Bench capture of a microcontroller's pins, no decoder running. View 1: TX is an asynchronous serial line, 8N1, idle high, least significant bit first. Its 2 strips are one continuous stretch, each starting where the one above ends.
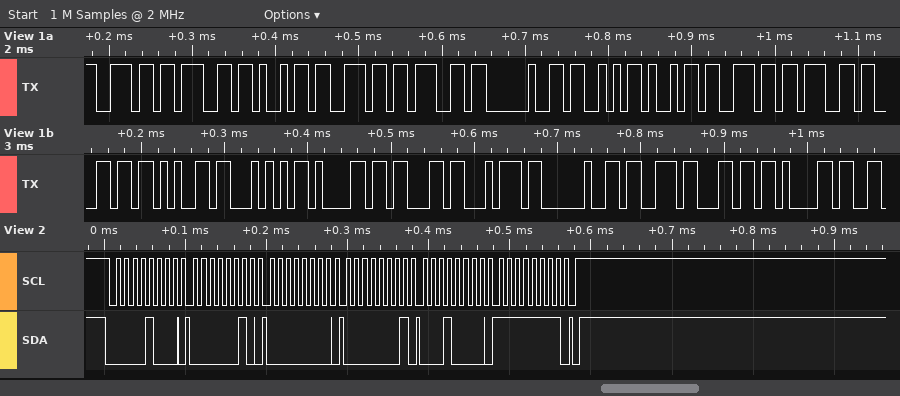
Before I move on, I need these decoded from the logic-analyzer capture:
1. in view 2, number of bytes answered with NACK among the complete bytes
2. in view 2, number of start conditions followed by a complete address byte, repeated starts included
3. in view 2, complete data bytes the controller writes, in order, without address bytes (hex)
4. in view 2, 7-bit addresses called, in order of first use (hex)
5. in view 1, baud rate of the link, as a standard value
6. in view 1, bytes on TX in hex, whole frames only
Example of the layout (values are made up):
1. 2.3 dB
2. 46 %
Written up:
1. 0
2. 1
3. 02 00 01 10 FF
4. 0x04
5. 115200 baud
6. 6E 67 69 6E 67 20 53 69 6E 67 6C 65 54 61 63 74 20 73 6C 61
